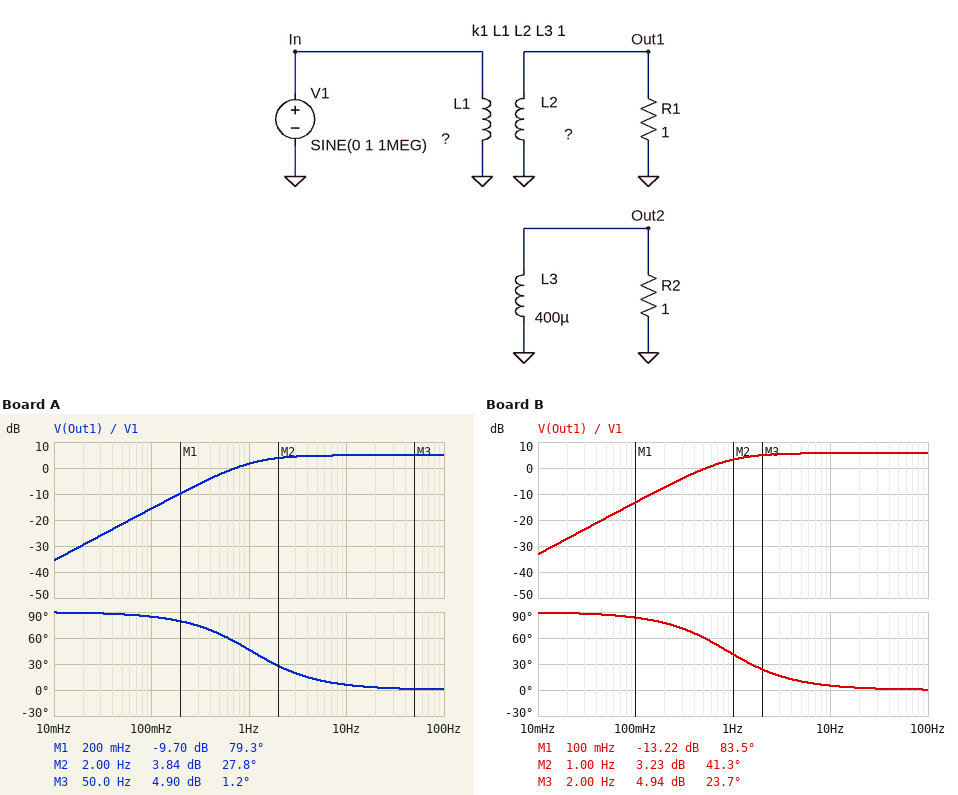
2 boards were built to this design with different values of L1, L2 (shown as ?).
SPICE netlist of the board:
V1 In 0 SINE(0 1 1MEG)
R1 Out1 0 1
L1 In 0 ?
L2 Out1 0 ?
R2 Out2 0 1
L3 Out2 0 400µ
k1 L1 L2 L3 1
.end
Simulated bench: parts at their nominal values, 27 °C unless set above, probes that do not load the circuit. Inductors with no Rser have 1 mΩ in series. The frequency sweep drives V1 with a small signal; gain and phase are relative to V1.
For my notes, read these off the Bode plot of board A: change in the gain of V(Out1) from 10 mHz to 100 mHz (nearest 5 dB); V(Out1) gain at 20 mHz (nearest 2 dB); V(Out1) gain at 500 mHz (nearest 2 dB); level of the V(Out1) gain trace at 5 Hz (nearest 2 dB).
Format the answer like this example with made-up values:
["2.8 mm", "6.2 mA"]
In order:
["20 dB", "-30 dB", "-2 dB", "4 dB"]
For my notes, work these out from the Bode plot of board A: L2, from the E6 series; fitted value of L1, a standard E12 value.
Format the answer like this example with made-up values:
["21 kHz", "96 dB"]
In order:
["470 µH", "150 µH"]
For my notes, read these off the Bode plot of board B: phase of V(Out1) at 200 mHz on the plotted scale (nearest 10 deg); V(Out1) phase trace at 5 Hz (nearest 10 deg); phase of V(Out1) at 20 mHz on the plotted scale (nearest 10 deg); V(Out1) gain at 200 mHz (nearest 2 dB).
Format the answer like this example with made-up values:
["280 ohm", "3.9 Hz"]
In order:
["80 deg", "10 deg", "90 deg", "-8 dB"]
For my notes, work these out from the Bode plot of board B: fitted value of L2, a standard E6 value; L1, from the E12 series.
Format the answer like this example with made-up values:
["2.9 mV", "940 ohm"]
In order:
["680 µH", "180 µH"]
